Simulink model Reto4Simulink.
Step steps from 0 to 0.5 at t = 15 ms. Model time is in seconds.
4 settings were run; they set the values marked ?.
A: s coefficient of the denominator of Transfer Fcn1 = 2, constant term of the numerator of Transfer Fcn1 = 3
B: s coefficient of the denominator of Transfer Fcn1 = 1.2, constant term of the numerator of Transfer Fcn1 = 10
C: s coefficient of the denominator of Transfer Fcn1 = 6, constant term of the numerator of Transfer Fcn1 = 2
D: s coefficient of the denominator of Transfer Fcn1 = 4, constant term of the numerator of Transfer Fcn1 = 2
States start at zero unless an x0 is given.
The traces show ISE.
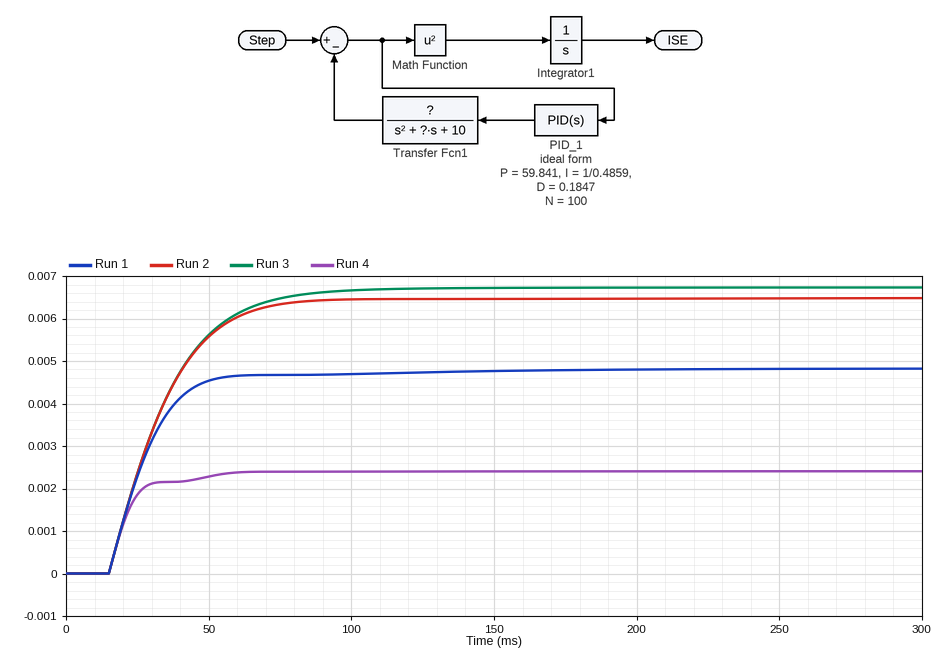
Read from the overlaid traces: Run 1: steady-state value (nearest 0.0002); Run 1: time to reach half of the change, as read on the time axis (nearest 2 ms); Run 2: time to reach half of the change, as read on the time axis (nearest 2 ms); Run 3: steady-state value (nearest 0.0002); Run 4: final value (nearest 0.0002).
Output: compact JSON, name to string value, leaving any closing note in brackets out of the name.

{"Run 1: steady-state value": "0.0048", "Run 1: time to reach half of the change, as read on the time axis": "26 ms", "Run 2: time to reach half of the change, as read on the time axis": "30 ms", "Run 3: steady-state value": "0.0068", "Run 4: final value": "0.0024"}
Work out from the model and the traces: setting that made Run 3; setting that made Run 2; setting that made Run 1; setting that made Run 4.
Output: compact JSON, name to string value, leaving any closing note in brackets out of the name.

{"setting that made Run 3": "C", "setting that made Run 2": "D", "setting that made Run 1": "A", "setting that made Run 4": "B"}
